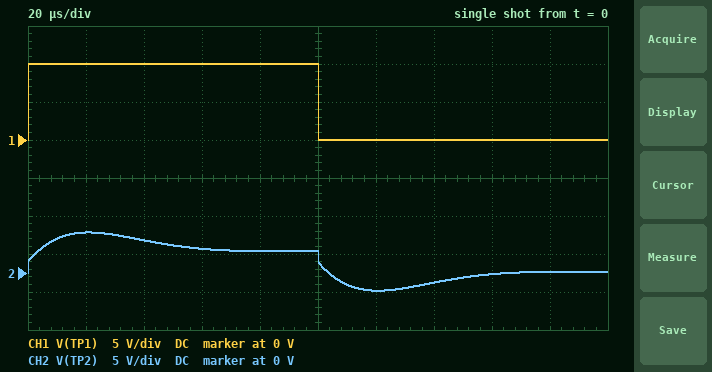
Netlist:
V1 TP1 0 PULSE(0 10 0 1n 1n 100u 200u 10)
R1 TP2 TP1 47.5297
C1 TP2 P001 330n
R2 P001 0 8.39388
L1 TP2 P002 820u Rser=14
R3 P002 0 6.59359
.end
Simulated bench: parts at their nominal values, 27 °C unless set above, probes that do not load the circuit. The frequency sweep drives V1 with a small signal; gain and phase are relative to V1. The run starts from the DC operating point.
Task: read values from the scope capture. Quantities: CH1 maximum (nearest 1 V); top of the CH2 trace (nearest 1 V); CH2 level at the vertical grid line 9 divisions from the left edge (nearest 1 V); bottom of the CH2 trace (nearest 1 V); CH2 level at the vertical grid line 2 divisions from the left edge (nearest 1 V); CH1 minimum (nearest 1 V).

10 V
5 V
0 V
-2 V
4 V
0 V
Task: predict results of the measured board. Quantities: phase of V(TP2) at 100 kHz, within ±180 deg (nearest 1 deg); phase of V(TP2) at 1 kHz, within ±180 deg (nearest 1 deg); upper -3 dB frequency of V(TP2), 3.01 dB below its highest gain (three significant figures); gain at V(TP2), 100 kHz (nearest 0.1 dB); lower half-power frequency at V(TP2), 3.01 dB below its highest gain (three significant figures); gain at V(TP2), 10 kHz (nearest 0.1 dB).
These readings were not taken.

-24 deg
8 deg
19.6 kHz
-15.2 dB
4.73 kHz
-3.5 dB
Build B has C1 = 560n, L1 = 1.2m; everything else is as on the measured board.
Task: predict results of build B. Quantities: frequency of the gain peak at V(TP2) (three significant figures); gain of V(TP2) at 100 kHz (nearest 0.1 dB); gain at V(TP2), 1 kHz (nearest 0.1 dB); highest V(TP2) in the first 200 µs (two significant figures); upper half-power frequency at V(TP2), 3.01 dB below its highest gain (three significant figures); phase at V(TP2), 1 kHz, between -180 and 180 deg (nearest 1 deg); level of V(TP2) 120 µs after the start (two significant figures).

6.45 kHz
-16.0 dB
-9.8 dB
5.1 V
12.3 kHz
11 deg
-1.8 V
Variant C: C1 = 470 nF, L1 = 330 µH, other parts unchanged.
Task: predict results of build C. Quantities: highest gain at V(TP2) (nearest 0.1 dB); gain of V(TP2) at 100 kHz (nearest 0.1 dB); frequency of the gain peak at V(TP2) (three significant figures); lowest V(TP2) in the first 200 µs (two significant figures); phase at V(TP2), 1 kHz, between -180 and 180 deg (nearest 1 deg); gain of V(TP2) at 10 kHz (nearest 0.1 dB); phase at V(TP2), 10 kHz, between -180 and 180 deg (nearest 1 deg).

-7.7 dB
-15.8 dB
12.0 kHz
-740 mV
2 deg
-7.9 dB
-4 deg
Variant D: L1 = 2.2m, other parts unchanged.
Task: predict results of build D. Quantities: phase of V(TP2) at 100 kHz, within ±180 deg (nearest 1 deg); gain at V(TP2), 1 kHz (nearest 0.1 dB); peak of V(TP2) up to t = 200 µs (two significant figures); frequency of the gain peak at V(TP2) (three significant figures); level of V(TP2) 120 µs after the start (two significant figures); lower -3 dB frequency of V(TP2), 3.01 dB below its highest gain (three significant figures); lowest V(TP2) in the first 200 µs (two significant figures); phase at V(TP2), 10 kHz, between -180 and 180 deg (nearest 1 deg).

-25 deg
-8.8 dB
6.7 V
6.35 kHz
-3.2 V
2.75 kHz
-3.6 V
-27 deg
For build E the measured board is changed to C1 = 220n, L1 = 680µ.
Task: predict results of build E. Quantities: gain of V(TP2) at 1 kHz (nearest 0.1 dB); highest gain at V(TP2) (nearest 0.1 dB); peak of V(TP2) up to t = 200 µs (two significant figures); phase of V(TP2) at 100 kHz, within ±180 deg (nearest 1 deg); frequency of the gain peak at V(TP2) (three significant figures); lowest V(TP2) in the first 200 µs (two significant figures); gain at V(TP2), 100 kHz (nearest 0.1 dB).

-10.2 dB
-2.9 dB
5.6 V
-32 deg
13.8 kHz
-2.6 V
-14.0 dB
